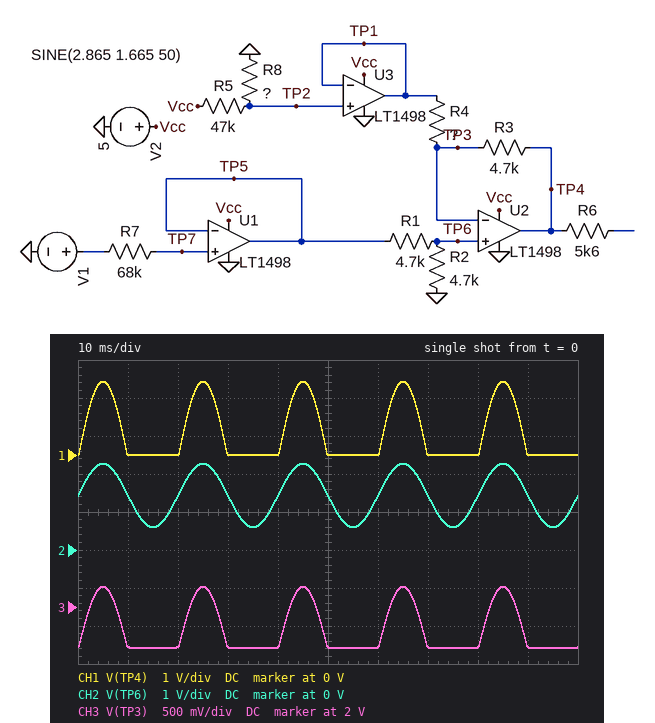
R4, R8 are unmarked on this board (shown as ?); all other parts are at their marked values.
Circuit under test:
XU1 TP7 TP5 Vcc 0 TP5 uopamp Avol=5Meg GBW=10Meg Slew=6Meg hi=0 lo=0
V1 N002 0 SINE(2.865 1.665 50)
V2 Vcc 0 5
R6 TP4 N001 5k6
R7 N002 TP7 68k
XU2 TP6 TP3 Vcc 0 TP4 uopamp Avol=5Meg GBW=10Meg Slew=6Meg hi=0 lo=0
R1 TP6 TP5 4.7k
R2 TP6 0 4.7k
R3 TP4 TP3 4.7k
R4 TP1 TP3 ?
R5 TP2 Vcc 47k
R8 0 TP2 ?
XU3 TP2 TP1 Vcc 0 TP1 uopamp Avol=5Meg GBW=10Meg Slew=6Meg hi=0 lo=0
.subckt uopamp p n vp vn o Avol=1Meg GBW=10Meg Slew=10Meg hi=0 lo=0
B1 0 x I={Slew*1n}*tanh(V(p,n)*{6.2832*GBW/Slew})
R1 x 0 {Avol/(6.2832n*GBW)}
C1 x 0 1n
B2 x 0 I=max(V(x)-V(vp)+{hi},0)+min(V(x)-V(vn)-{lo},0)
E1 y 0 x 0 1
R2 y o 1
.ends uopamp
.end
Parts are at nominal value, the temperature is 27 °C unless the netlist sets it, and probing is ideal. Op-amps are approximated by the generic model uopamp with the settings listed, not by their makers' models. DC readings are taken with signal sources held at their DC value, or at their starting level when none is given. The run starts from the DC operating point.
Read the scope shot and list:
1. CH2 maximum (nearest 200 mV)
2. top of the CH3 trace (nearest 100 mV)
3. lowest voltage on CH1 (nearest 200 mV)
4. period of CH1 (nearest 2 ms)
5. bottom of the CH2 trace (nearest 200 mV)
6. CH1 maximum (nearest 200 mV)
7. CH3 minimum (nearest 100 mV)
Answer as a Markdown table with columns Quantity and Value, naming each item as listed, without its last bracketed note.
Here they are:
| Quantity | Value |
|---|---|
| CH2 maximum | 2.2 V |
| top of the CH3 trace | 2.3 V |
| lowest voltage on CH1 | 0 V |
| period of CH1 | 20 ms |
| bottom of the CH2 trace | 600 mV |
| CH1 maximum | 2.0 V |
| CH3 minimum | 1.5 V |
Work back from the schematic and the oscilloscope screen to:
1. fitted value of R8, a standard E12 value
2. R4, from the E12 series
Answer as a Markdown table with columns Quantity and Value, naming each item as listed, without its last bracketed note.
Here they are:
| Quantity | Value |
|---|---|
| fitted value of R8, a standard E12 value | 47 kΩ |
| R4, from the E12 series | 3.3 kΩ |
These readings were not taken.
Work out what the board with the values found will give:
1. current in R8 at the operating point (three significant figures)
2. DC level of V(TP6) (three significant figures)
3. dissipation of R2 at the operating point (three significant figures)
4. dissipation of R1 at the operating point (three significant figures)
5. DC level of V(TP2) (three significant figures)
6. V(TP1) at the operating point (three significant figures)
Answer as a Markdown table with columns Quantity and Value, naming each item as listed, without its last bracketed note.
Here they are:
| Quantity | Value |
|---|---|
| current in R8 at the operating point | 53.2 µA |
| DC level of V(TP6) | 1.43 V |
| dissipation of R2 at the operating point | 437 µW |
| dissipation of R1 at the operating point | 437 µW |
| DC level of V(TP2) | 2.50 V |
| V(TP1) at the operating point | 2.50 V |
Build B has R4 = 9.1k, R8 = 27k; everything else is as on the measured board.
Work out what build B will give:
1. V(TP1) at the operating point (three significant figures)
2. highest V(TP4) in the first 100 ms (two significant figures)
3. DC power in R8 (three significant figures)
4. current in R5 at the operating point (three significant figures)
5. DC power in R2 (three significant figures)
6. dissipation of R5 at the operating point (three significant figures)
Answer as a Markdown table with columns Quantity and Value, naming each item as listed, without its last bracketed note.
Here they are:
| Quantity | Value |
|---|---|
| V(TP1) at the operating point | 1.82 V |
| highest V(TP4) in the first 100 ms | 2.5 V |
| DC power in R8 | 123 µW |
| current in R5 at the operating point | 67.6 µA |
| DC power in R2 | 437 µW |
| dissipation of R5 at the operating point | 215 µW |
